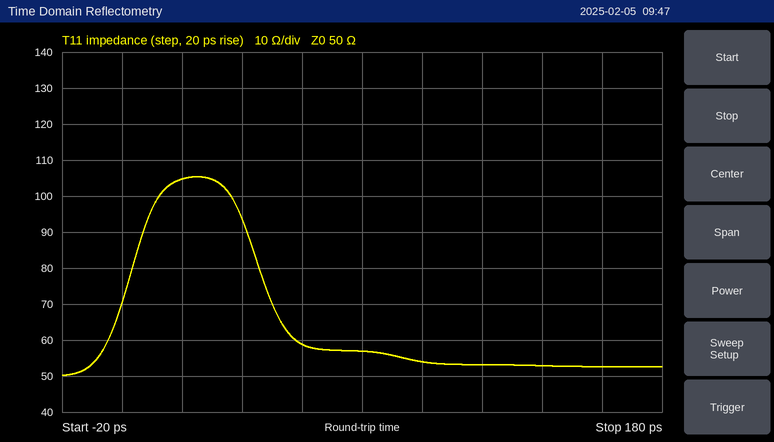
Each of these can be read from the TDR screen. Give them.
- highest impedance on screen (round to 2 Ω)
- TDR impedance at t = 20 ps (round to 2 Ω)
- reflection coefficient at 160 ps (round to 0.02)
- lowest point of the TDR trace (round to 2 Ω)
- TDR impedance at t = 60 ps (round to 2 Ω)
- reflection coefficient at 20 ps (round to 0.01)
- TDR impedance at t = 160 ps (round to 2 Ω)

106 Ω
104 Ω
+0.02
50 Ω
58 Ω
+0.35
52 Ω
